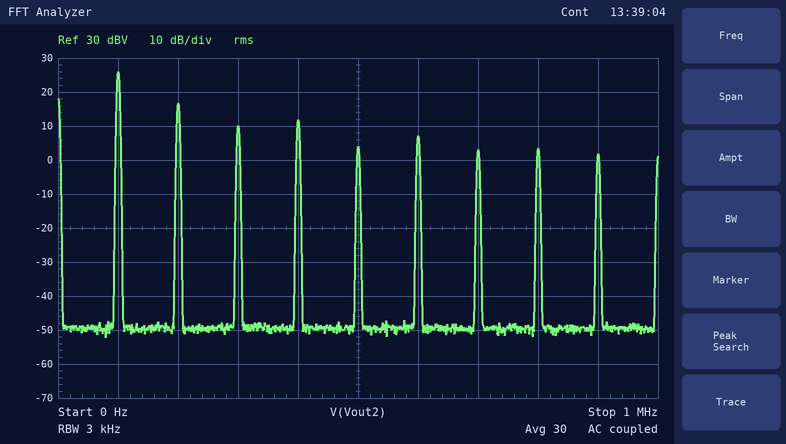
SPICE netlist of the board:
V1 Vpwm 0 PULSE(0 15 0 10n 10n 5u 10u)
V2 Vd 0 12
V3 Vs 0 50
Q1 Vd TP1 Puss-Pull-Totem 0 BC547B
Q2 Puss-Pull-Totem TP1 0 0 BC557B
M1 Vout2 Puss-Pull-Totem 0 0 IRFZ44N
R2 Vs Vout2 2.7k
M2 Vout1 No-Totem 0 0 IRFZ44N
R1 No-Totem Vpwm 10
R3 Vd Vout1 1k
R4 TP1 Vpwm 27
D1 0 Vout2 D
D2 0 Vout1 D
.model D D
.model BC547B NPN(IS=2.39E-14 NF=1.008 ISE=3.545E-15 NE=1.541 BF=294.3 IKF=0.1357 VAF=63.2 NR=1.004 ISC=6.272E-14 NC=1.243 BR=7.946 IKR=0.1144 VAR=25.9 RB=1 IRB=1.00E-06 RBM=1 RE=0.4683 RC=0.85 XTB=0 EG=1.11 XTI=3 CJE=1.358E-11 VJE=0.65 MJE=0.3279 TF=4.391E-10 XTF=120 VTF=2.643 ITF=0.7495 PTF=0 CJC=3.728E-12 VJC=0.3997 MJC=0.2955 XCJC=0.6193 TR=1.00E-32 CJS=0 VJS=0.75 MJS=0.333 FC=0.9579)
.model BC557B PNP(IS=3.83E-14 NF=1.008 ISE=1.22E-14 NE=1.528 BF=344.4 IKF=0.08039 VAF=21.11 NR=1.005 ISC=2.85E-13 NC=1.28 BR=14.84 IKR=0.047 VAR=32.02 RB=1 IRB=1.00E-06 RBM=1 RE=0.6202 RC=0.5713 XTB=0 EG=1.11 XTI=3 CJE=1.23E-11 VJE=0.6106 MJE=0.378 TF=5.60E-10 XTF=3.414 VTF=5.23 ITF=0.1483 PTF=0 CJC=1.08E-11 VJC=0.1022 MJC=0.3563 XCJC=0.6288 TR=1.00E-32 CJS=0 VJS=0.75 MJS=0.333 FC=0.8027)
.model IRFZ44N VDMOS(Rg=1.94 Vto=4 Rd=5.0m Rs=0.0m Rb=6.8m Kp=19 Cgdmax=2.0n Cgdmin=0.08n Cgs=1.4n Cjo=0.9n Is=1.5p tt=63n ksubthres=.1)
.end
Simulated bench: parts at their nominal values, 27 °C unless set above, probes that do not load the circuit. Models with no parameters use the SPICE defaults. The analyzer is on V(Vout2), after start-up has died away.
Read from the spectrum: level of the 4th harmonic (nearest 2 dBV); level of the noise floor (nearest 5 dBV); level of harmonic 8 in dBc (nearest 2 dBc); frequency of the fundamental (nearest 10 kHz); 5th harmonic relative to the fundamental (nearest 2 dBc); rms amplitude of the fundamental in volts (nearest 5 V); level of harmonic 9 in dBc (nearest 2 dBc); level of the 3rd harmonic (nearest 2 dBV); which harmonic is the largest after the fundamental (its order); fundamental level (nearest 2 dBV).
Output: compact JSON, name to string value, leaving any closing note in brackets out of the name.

{"level of the 4th harmonic": "12 dBV", "level of the noise floor": "-50 dBV", "level of harmonic 8 in dBc": "-22 dBc", "frequency of the fundamental": "100 kHz", "5th harmonic relative to the fundamental": "-22 dBc", "rms amplitude of the fundamental in volts": "20 V", "level of harmonic 9 in dBc": "-24 dBc", "level of the 3rd harmonic": "10 dBV", "which harmonic is the largest after the fundamental": "2", "fundamental level": "26 dBV"}
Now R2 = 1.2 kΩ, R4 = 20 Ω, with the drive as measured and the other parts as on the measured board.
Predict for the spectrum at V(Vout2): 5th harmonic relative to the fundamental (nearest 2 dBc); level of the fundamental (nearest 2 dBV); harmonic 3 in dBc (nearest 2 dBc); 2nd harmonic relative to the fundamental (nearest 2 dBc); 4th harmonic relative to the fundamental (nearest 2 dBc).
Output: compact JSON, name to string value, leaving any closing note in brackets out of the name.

{"5th harmonic relative to the fundamental": "-20 dBc", "level of the fundamental": "26 dBV", "harmonic 3 in dBc": "-12 dBc", "2nd harmonic relative to the fundamental": "-14 dBc", "4th harmonic relative to the fundamental": "-16 dBc"}
